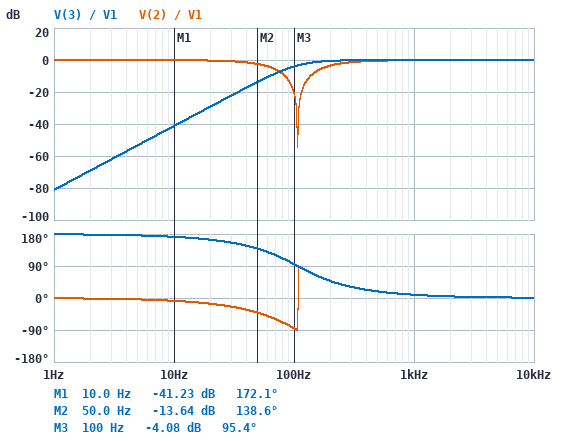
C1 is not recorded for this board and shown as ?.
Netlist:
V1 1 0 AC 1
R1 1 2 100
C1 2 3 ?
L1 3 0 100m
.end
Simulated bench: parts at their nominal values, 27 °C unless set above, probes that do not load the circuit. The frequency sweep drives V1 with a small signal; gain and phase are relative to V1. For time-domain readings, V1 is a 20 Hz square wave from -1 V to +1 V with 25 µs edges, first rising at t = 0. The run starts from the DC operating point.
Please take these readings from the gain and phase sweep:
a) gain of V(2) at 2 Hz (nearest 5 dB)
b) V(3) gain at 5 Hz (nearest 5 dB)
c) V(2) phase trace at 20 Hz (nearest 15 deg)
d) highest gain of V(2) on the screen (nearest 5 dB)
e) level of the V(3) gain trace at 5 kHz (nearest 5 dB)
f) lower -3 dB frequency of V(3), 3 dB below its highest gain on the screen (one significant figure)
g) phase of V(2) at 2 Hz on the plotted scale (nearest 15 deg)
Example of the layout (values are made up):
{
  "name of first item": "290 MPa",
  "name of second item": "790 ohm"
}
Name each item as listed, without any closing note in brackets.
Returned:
{
  "gain of V(2) at 2 Hz": "0 dB",
  "V(3) gain at 5 Hz": "-55 dB",
  "V(2) phase trace at 20 Hz": "-15 deg",
  "highest gain of V(2) on the screen": "0 dB",
  "level of the V(3) gain trace at 5 kHz": "0 dB",
  "lower -3 dB frequency of V(3), 3 dB below its highest gain on the screen": "100 Hz",
  "phase of V(2) at 2 Hz on the plotted scale": "0 deg"
}
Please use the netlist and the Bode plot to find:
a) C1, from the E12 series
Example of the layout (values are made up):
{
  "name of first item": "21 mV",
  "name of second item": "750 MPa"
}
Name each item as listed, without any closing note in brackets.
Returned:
{
  "C1, from the E12 series": "22 µF"
}
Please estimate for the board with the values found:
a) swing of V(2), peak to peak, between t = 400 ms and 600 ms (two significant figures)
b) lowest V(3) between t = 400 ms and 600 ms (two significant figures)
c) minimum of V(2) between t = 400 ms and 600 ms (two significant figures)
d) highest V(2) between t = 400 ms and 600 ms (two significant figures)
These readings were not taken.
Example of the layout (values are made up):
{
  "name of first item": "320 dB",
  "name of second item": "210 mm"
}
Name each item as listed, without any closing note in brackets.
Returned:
{
  "swing of V(2), peak to peak, between t = 400 ms and 600 ms": "2.1 V",
  "lowest V(3) between t = 400 ms and 600 ms": "-2.0 V",
  "minimum of V(2) between t = 400 ms and 600 ms": "-1.0 V",
  "highest V(2) between t = 400 ms and 600 ms": "1.0 V"
}
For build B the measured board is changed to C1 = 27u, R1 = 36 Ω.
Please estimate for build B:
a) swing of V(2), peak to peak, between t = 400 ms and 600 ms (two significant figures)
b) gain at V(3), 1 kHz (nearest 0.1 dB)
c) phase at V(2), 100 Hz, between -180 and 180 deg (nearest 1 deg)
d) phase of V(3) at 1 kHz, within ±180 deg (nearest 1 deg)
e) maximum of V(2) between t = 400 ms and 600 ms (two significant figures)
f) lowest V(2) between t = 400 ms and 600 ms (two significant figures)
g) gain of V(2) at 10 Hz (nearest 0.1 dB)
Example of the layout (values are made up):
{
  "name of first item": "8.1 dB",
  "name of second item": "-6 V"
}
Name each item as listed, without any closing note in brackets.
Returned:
{
  "swing of V(2), peak to peak, between t = 400 ms and 600 ms": "2.6 V",
  "gain at V(3), 1 kHz": "0.1 dB",
  "phase at V(2), 100 Hz, between -180 and 180 deg": "84 deg",
  "phase of V(3) at 1 kHz, within ±180 deg": "3 deg",
  "maximum of V(2) between t = 400 ms and 600 ms": "1.3 V",
  "lowest V(2) between t = 400 ms and 600 ms": "-1.3 V",
  "gain of V(2) at 10 Hz": "0 dB"
}
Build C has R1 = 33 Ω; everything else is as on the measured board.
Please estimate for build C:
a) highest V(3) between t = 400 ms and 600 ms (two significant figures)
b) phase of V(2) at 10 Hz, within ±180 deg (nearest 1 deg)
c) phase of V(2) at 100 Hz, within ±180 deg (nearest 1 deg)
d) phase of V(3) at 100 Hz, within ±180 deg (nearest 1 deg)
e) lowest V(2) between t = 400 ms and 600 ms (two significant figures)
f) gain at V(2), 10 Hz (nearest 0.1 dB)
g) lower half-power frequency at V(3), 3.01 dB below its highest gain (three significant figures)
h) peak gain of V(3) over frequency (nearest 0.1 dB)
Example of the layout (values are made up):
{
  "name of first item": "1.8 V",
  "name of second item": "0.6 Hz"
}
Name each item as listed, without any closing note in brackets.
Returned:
{
  "highest V(3) between t = 400 ms and 600 ms": "2.0 V",
  "phase of V(2) at 10 Hz, within ±180 deg": "-3 deg",
  "phase of V(2) at 100 Hz, within ±180 deg": "-74 deg",
  "phase of V(3) at 100 Hz, within ±180 deg": "106 deg",
  "lowest V(2) between t = 400 ms and 600 ms": "-1.3 V",
  "gain at V(2), 10 Hz": "0 dB",
  "lower half-power frequency at V(3), 3.01 dB below its highest gain": "92.2 Hz",
  "peak gain of V(3) over frequency": "6.5 dB"
}
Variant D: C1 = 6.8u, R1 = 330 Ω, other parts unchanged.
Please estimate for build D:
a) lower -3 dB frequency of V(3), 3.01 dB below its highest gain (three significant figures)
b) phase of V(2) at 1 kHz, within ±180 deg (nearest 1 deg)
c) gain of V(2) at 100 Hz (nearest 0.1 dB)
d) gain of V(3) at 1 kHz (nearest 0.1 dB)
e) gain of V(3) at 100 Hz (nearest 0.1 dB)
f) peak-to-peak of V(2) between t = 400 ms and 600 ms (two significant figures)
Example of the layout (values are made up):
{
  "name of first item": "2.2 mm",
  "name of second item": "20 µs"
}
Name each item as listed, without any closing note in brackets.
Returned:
{
  "lower -3 dB frequency of V(3), 3.01 dB below its highest gain": "456 Hz",
  "phase of V(2) at 1 kHz, within ±180 deg": "29 deg",
  "gain of V(2) at 100 Hz": "-6.7 dB",
  "gain of V(3) at 1 kHz": "-0.8 dB",
  "gain of V(3) at 100 Hz": "-15.4 dB",
  "peak-to-peak of V(2) between t = 400 ms and 600 ms": "2.0 V"
}
